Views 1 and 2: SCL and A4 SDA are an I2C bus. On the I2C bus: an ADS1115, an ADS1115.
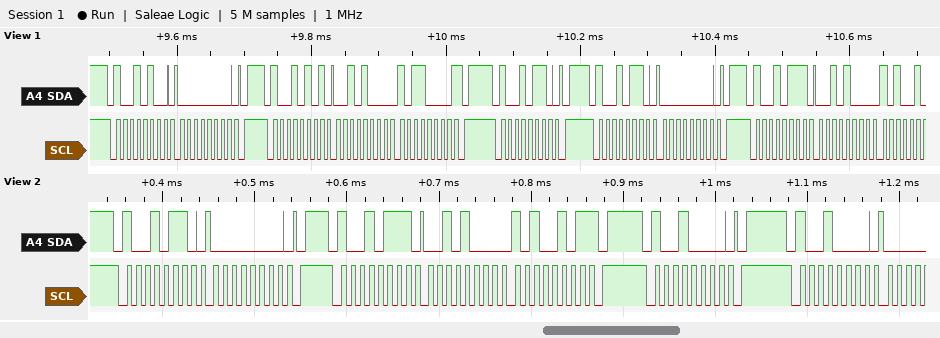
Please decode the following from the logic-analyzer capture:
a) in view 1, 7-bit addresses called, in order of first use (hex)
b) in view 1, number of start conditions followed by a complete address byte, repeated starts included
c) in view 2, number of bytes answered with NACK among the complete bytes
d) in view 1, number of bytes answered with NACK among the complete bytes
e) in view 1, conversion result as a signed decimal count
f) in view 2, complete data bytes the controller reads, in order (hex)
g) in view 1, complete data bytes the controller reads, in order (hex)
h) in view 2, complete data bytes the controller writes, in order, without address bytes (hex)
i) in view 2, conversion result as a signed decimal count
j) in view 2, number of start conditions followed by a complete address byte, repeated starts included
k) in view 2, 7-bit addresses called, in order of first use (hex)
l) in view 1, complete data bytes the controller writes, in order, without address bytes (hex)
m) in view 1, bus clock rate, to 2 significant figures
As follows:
0x4A 0x4B
5
1
1
10416
28 A5
28 B0 28
00
10405
4
0x4B 0x48
00 00
100 kHz
